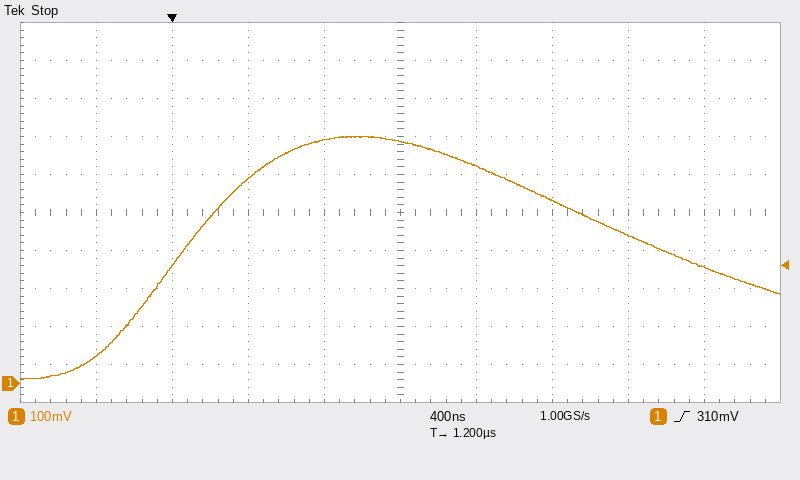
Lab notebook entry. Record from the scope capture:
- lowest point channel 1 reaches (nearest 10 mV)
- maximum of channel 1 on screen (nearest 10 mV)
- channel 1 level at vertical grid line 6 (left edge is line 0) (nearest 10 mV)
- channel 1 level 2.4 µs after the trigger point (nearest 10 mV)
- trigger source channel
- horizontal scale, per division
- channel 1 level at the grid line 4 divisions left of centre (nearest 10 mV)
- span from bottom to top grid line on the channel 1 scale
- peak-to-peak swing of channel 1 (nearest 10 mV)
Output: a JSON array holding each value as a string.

["10 mV", "650 mV", "570 mV", "390 mV", "channel 1", "400 ns", "70 mV", "1 V", "640 mV"]
